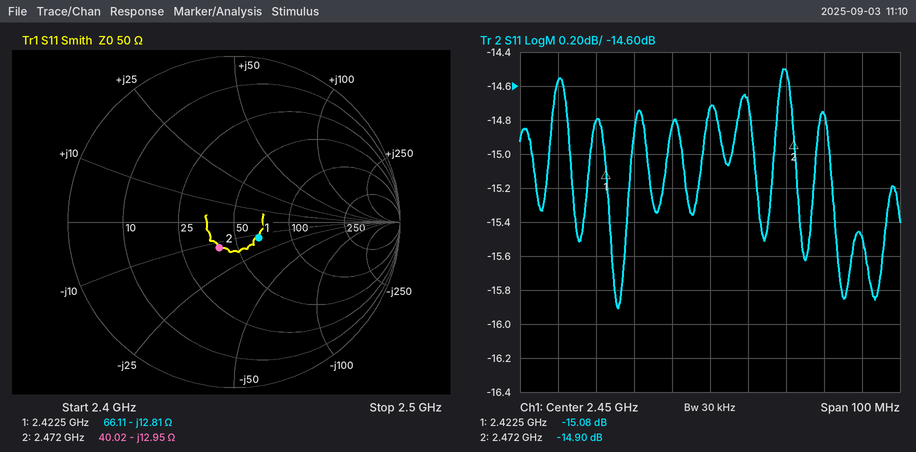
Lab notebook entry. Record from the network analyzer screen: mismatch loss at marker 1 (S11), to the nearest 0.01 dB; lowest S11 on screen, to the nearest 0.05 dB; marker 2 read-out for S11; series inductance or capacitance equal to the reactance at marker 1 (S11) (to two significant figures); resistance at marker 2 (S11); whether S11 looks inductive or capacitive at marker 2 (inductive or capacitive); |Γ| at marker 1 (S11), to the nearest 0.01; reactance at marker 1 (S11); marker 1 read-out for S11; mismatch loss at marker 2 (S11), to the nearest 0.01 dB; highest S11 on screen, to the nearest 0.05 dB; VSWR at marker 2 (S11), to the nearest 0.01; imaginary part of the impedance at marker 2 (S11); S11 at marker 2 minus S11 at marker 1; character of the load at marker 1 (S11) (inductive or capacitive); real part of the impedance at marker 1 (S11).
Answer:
0.14 dB
-15.90 dB
-14.90 dB
5.1 pF
40.02 Ω
capacitive
0.18
-12.81 Ω
-15.08 dB
0.14 dB
-14.50 dB
1.44
-12.95 Ω
0.18 dB
capacitive
66.11 Ω
